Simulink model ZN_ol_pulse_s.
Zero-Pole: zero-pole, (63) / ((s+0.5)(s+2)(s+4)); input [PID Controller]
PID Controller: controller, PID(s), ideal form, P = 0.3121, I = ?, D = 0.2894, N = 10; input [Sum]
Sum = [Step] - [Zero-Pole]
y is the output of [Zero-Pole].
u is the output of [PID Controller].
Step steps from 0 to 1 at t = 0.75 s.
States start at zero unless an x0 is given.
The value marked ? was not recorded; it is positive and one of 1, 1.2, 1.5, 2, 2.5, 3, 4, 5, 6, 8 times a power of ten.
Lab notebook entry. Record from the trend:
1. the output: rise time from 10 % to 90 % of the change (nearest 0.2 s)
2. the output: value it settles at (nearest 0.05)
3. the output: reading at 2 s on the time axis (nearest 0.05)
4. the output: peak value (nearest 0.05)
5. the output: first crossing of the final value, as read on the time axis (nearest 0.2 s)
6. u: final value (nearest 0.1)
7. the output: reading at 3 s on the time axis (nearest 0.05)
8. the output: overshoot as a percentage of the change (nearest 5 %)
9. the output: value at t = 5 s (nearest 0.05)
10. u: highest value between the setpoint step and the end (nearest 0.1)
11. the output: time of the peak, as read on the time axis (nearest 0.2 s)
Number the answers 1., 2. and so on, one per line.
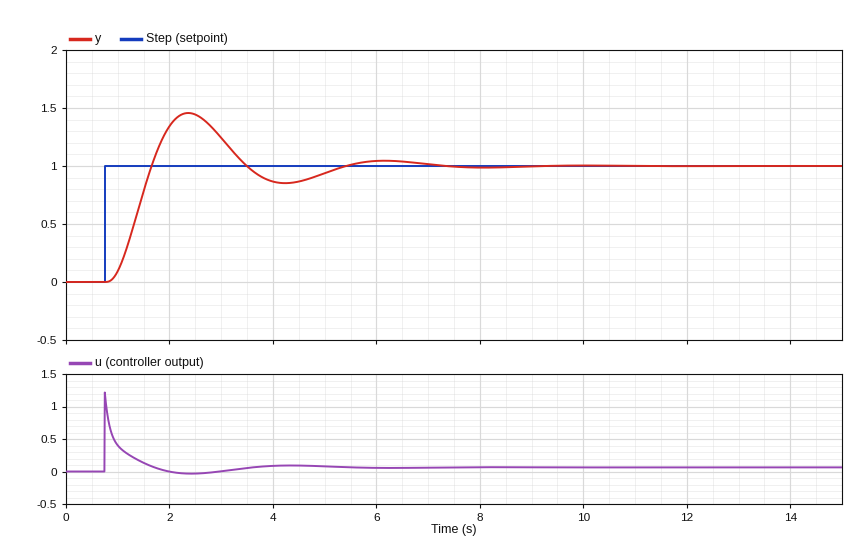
1. 0.6 s
2. 1.00
3. 1.35
4. 1.45
5. 1.6 s
6. 0.1
7. 1.25
8. 45 %
9. 0.95
10. 1.2
11. 2.4 s
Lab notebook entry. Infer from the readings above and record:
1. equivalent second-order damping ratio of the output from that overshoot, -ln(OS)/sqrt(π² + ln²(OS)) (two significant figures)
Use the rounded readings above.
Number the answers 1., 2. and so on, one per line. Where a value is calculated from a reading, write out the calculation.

1. ln(0.45) = -0.799; 0.799 / sqrt(9.870 + 0.638) = 0.25
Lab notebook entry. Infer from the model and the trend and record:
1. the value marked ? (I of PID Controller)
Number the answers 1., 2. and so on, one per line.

1. 1.2
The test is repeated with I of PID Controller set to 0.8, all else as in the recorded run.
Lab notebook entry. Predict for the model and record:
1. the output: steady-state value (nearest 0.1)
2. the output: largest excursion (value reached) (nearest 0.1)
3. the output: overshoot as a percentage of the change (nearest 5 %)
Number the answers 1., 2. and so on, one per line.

1. 1.0
2. 1.3
3. 30 %
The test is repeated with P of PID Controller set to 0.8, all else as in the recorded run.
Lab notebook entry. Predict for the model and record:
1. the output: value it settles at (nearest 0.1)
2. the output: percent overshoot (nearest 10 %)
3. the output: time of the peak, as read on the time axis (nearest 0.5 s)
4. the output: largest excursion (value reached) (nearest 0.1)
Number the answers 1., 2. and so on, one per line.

1. 1.0
2. 70 %
3. 1.5 s
4. 1.7
